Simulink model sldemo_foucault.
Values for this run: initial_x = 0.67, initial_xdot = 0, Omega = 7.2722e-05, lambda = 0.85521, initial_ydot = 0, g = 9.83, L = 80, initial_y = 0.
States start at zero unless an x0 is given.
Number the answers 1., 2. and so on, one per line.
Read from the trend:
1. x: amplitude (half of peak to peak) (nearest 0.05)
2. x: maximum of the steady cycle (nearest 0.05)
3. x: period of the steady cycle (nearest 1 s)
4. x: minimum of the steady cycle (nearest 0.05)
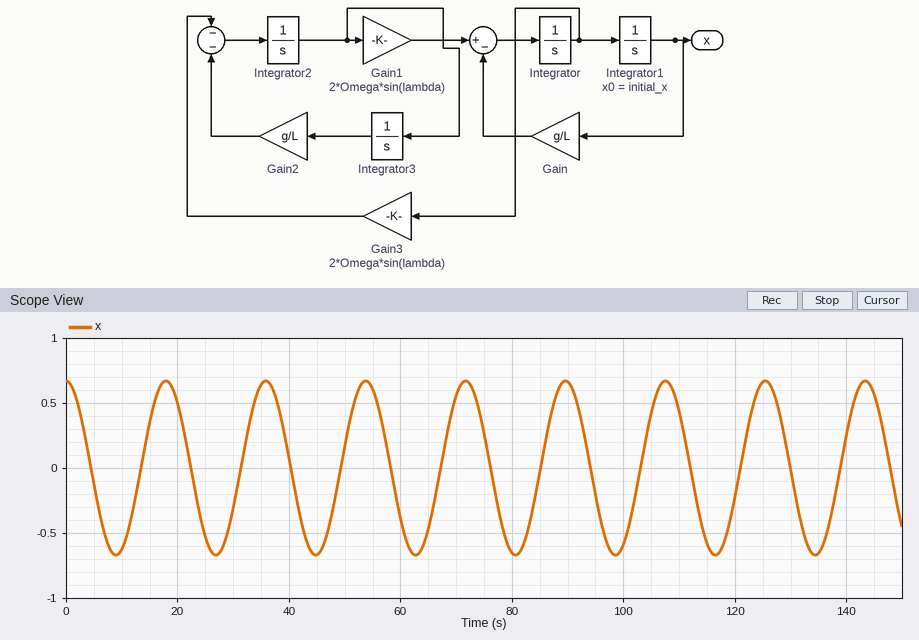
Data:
1. 0.65
2. 0.65
3. 18 s
4. -0.65
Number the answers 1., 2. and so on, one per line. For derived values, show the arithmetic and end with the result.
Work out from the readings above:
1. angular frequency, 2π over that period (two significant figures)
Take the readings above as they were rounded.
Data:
1. 2π / 18 = 0.35 rad/s
